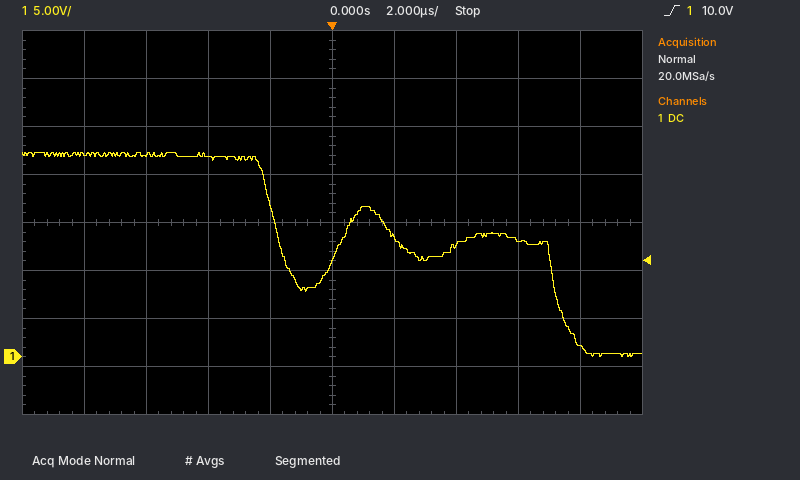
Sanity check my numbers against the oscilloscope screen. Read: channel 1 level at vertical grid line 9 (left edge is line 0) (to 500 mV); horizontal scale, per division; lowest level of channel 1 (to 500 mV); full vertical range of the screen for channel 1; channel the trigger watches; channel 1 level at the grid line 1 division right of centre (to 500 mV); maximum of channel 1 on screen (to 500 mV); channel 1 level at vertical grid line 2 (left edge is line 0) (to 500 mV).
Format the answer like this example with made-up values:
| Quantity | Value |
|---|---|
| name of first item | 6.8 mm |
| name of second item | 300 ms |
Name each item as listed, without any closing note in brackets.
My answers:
| Quantity | Value |
|---|---|
| channel 1 level at vertical grid line 9 (left edge is line 0) | 1.0 V |
| horizontal scale, per division | 2 µs |
| lowest level of channel 1 | 0.0 V |
| full vertical range of the screen for channel 1 | 40 V |
| channel the trigger watches | channel 1 |
| channel 1 level at the grid line 1 division right of centre | 12.5 V |
| maximum of channel 1 on screen | 21.5 V |
| channel 1 level at vertical grid line 2 (left edge is line 0) | 21.0 V |
